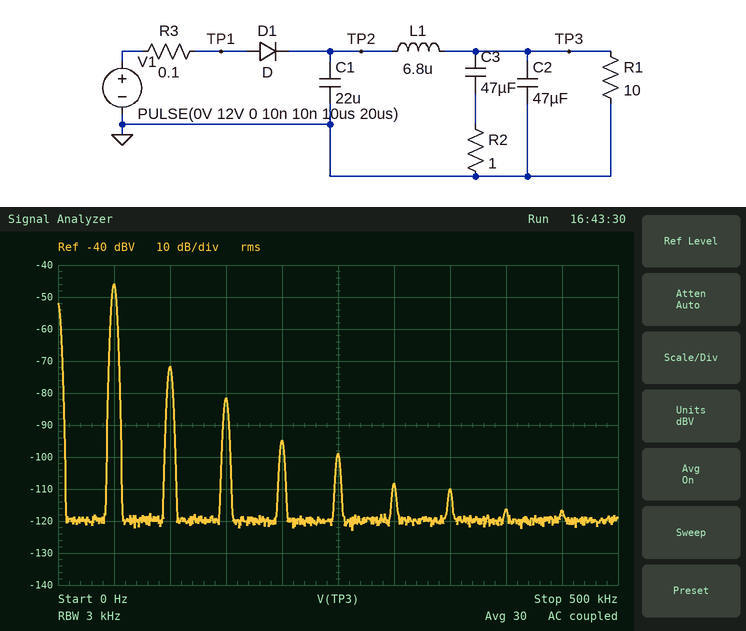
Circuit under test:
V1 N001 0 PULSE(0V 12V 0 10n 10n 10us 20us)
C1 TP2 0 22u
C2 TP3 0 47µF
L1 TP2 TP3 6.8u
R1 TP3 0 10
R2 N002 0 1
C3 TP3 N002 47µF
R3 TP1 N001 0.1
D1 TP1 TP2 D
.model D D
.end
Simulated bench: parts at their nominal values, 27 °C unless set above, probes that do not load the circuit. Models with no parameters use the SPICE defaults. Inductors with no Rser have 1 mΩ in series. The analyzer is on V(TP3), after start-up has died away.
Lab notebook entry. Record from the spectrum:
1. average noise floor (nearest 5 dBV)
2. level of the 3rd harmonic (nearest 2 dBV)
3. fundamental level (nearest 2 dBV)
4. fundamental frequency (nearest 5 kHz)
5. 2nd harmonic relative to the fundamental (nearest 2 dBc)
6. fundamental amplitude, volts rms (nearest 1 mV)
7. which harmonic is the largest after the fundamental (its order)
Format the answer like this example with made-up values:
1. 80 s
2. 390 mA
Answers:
1. -120 dBV
2. -82 dBV
3. -46 dBV
4. 50 kHz
5. -26 dBc
6. 5 mV
7. 2
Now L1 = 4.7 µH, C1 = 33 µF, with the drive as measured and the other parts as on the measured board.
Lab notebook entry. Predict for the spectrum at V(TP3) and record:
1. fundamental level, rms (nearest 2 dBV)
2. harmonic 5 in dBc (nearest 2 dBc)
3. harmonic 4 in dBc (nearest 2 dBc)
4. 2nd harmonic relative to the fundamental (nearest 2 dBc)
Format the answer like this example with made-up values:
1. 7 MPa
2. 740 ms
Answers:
1. -46 dBV
2. -54 dBc
3. -52 dBc
4. -28 dBc
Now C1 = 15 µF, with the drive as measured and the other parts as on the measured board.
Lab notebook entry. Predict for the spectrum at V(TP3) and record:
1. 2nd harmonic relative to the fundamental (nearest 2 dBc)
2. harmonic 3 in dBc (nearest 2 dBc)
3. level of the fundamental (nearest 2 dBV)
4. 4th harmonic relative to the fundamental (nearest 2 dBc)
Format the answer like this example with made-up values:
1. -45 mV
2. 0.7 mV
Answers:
1. -24 dBc
2. -34 dBc
3. -42 dBV
4. -46 dBc
